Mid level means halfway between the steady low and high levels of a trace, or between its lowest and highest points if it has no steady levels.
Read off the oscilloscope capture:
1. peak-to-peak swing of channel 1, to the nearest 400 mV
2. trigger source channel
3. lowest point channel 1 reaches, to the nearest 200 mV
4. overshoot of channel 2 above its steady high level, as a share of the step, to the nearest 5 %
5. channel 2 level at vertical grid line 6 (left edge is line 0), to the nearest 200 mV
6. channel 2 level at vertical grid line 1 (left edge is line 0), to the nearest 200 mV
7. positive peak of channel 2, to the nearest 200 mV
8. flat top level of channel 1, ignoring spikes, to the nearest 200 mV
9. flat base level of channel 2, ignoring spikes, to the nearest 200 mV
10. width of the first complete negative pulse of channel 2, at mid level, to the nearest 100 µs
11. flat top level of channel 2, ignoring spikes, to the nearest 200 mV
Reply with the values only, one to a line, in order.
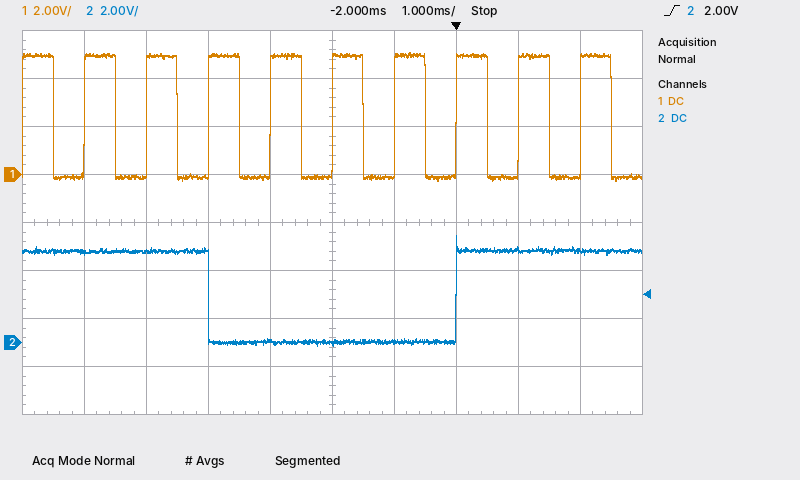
5.2 V
channel 2
-200 mV
15 %
0.0 V
3.8 V
4.4 V
5.0 V
0.0 V
4.0 ms
3.8 V
